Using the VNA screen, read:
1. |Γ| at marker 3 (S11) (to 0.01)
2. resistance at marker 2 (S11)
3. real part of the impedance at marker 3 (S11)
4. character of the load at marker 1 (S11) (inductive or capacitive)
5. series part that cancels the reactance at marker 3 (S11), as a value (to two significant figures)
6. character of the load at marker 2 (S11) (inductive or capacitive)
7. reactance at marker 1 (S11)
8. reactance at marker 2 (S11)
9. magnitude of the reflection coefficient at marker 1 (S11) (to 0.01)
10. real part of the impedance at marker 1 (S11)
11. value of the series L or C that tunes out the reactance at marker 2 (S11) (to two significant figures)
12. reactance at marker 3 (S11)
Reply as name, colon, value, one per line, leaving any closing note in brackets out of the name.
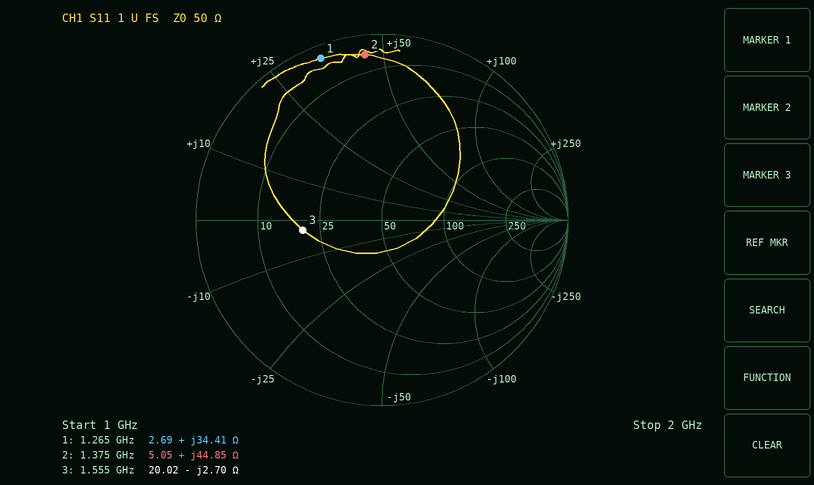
|Γ| at marker 3 (S11): 0.43
resistance at marker 2: 5.05 Ω
real part of the impedance at marker 3: 20.02 Ω
character of the load at marker 1 (S11): inductive
series part that cancels the reactance at marker 3 (S11), as a value: 280 pH
character of the load at marker 2 (S11): inductive
reactance at marker 1: +34.41 Ω
reactance at marker 2: +44.85 Ω
magnitude of the reflection coefficient at marker 1 (S11): 0.93
real part of the impedance at marker 1: 2.69 Ω
value of the series L or C that tunes out the reactance at marker 2 (S11): 2.6 pF
reactance at marker 3: -2.70 Ω
